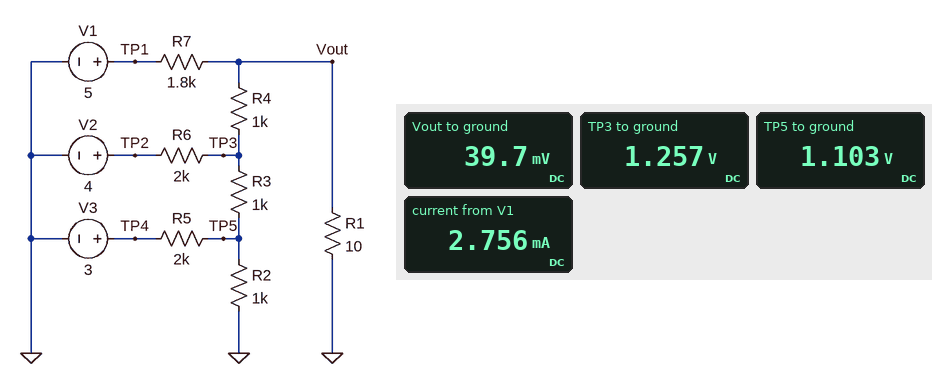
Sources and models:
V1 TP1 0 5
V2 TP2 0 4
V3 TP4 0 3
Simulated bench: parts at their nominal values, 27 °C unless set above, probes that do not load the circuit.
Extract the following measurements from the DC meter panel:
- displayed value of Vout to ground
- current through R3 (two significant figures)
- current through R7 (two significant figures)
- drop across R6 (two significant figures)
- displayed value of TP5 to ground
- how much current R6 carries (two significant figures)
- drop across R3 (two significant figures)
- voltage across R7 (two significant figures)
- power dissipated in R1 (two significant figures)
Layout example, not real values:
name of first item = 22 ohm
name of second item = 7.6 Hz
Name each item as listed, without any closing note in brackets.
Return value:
displayed value of Vout to ground = 39.7 mV
current through R3 = 150 µA
current through R7 = 2.8 mA
drop across R6 = 2.7 V
displayed value of TP5 to ground = 1.103 V
how much current R6 carries = 1.4 mA
drop across R3 = 150 mV
voltage across R7 = 5.0 V
power dissipated in R1 = 160 µW
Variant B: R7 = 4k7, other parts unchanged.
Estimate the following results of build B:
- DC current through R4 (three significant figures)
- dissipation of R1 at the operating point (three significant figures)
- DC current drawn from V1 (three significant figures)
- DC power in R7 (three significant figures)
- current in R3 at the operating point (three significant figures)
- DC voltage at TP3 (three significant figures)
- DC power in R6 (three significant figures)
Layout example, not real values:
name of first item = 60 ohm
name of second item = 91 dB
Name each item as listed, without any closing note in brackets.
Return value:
DC current through R4 = 1.23 mA
dissipation of R1 at the operating point = 52.2 µW
DC current drawn from V1 = 1.06 mA
DC power in R7 = 5.27 mW
current in R3 at the operating point = 149 µA
DC voltage at TP3 = 1.25 V
DC power in R6 = 3.78 mW
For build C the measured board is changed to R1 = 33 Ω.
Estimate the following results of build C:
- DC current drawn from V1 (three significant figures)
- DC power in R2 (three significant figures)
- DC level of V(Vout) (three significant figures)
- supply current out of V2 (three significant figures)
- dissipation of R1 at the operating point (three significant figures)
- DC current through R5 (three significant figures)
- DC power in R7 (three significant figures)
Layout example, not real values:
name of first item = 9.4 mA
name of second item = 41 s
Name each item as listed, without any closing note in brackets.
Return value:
DC current drawn from V1 = 2.71 mA
DC power in R2 = 1.25 mW
DC level of V(Vout) = 128 mV
supply current out of V2 = 1.35 mA
dissipation of R1 at the operating point = 496 µW
DC current through R5 = 940 µA
DC power in R7 = 13.2 mW
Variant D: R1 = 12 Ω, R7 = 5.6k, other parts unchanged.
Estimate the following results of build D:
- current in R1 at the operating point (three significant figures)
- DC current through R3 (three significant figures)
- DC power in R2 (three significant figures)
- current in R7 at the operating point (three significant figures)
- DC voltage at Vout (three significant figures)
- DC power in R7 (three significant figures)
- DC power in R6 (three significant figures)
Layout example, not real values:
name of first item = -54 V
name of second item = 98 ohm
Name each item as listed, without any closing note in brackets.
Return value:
current in R1 at the operating point = 2.11 mA
DC current through R3 = 150 µA
DC power in R2 = 1.21 mW
current in R7 at the operating point = 888 µA
DC voltage at Vout = 25.4 mV
DC power in R7 = 4.42 mW
DC power in R6 = 3.78 mW
